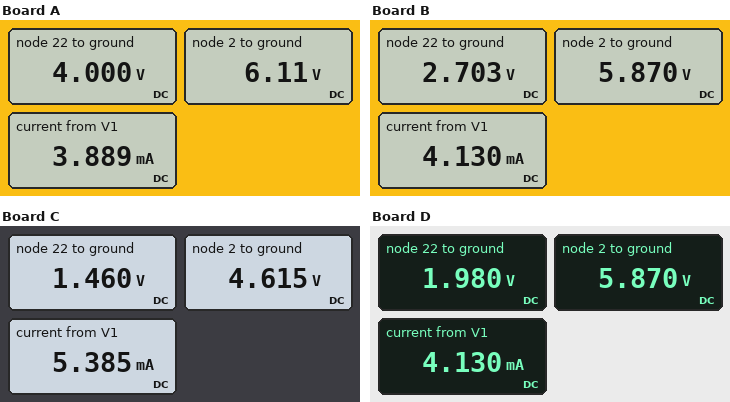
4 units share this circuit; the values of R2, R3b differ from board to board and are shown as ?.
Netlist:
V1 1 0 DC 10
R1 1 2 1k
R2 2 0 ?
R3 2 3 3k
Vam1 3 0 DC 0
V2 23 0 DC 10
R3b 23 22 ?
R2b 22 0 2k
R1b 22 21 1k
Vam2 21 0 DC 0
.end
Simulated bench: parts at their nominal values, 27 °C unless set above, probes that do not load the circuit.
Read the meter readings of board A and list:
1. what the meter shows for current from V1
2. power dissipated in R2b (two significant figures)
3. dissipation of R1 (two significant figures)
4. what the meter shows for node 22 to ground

3.889 mA
8.0 mW
15 mW
4.000 V
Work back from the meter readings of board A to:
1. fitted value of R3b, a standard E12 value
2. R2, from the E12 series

1 kΩ
3.3 kΩ
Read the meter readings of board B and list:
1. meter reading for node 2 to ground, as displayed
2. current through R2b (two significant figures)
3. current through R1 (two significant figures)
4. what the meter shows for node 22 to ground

5.870 V
1.4 mA
4.1 mA
2.703 V
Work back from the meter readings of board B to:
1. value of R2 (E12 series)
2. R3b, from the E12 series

2.7 kΩ
1.8 kΩ
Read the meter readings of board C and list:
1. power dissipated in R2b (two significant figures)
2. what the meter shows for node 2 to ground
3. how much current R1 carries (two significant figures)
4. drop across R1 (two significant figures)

1.1 mW
4.615 V
5.4 mA
5.4 V
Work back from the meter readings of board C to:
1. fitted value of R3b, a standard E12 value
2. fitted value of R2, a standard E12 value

3.9 kΩ
1.2 kΩ
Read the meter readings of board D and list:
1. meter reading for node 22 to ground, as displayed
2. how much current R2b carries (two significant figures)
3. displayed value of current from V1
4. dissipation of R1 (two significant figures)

1.980 V
990 µA
4.130 mA
17 mW
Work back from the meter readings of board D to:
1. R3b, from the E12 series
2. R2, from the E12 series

2.7 kΩ
2.7 kΩ
